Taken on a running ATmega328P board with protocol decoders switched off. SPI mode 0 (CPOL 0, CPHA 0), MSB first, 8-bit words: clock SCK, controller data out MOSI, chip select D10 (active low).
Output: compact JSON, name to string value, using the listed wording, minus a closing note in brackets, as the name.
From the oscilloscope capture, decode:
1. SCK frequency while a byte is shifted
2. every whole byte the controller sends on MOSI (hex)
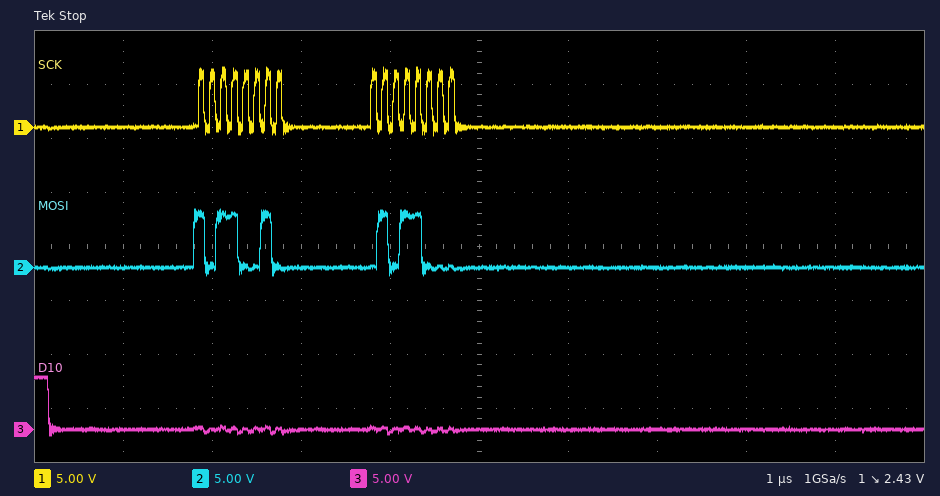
{"SCK frequency while a byte is shifted": "8 MHz", "every whole byte the controller sends on MOSI": "B2 58"}
